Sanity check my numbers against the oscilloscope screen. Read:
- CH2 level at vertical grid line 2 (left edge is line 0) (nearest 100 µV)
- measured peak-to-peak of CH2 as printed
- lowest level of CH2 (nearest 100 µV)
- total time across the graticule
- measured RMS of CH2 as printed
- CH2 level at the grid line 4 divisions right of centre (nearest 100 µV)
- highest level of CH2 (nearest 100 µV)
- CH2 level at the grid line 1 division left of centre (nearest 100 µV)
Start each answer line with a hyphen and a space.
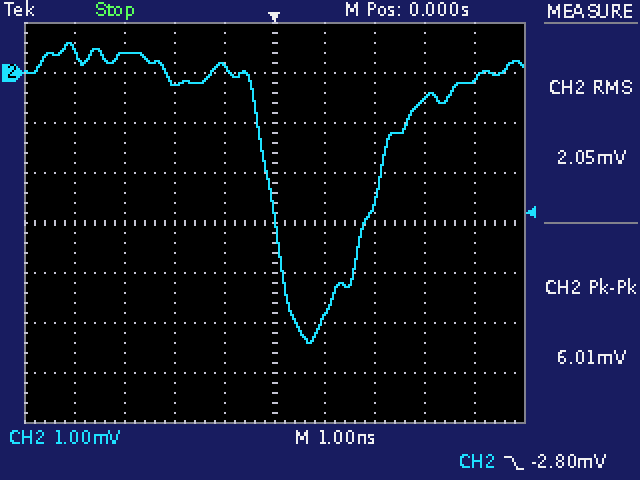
- 400 µV
- 6.01 mV
- -5.4 mV
- 10 ns
- 2.05 mV
- -100 µV
- 600 µV
- 100 µV
